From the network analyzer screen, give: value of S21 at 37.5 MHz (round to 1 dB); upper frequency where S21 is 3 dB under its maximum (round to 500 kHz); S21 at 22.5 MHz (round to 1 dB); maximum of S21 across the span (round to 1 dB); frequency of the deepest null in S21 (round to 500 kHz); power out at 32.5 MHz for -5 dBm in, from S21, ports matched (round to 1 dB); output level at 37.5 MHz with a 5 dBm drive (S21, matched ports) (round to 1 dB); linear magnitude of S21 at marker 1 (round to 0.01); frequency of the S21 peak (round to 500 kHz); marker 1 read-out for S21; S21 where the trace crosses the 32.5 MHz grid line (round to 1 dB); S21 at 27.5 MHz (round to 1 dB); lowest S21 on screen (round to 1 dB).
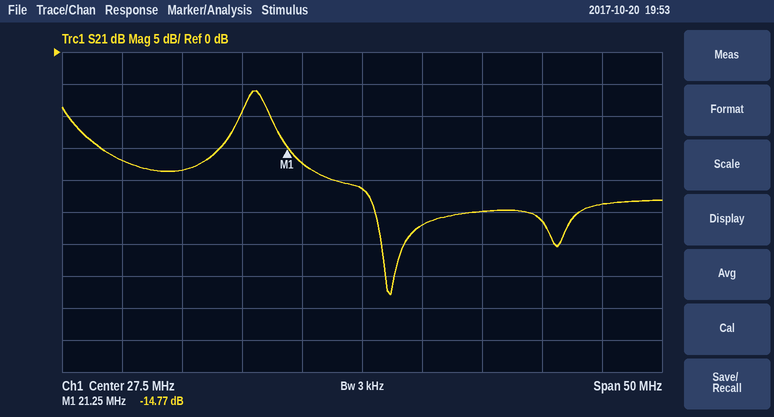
-25 dB
19.5 MHz
-17 dB
-6 dB
30.0 MHz
-32 dBm
-20 dBm
0.18
18.5 MHz
-14.77 dB
-27 dB
-21 dB
-38 dB
